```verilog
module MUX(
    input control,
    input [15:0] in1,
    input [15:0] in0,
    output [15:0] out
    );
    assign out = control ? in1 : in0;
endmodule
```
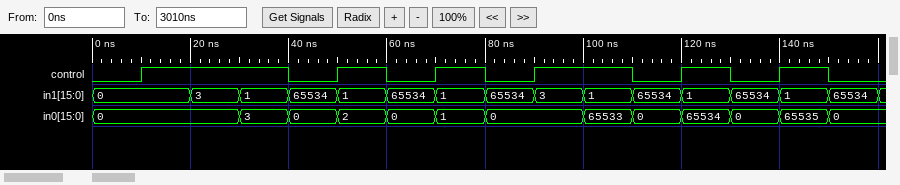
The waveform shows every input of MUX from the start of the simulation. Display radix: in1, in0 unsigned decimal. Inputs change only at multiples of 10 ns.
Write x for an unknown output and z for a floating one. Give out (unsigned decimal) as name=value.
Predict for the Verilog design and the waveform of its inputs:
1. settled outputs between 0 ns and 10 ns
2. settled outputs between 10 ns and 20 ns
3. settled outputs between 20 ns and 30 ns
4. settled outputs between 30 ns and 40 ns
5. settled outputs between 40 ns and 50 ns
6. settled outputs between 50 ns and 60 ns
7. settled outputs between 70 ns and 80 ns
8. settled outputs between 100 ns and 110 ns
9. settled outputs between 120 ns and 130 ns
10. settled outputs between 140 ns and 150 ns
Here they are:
out=0
out=0
out=3
out=1
out=0
out=1
out=1
out=1
out=1
out=1
